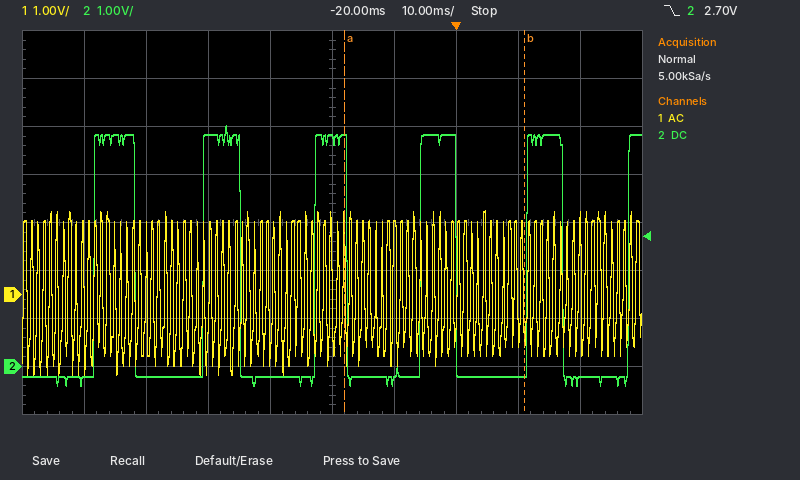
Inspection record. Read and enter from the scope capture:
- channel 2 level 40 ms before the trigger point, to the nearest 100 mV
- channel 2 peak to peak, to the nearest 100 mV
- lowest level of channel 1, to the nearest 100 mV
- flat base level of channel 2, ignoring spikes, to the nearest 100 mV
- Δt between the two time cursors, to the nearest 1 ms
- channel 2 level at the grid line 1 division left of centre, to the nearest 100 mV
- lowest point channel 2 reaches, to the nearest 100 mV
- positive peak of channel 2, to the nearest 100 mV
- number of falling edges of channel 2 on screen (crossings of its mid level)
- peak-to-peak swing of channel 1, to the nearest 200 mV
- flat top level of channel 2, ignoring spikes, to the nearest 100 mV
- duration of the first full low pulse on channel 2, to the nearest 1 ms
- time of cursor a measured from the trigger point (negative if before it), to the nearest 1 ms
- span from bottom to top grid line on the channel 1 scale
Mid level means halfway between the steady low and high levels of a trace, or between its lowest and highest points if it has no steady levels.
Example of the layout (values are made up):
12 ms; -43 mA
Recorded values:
4.8 V; 5.4 V; -1.7 V; -200 mV; 29 ms; -200 mV; -400 mV; 5.0 V; 5; 3.4 V; 4.8 V; 11 ms; -18 ms; 8 V
